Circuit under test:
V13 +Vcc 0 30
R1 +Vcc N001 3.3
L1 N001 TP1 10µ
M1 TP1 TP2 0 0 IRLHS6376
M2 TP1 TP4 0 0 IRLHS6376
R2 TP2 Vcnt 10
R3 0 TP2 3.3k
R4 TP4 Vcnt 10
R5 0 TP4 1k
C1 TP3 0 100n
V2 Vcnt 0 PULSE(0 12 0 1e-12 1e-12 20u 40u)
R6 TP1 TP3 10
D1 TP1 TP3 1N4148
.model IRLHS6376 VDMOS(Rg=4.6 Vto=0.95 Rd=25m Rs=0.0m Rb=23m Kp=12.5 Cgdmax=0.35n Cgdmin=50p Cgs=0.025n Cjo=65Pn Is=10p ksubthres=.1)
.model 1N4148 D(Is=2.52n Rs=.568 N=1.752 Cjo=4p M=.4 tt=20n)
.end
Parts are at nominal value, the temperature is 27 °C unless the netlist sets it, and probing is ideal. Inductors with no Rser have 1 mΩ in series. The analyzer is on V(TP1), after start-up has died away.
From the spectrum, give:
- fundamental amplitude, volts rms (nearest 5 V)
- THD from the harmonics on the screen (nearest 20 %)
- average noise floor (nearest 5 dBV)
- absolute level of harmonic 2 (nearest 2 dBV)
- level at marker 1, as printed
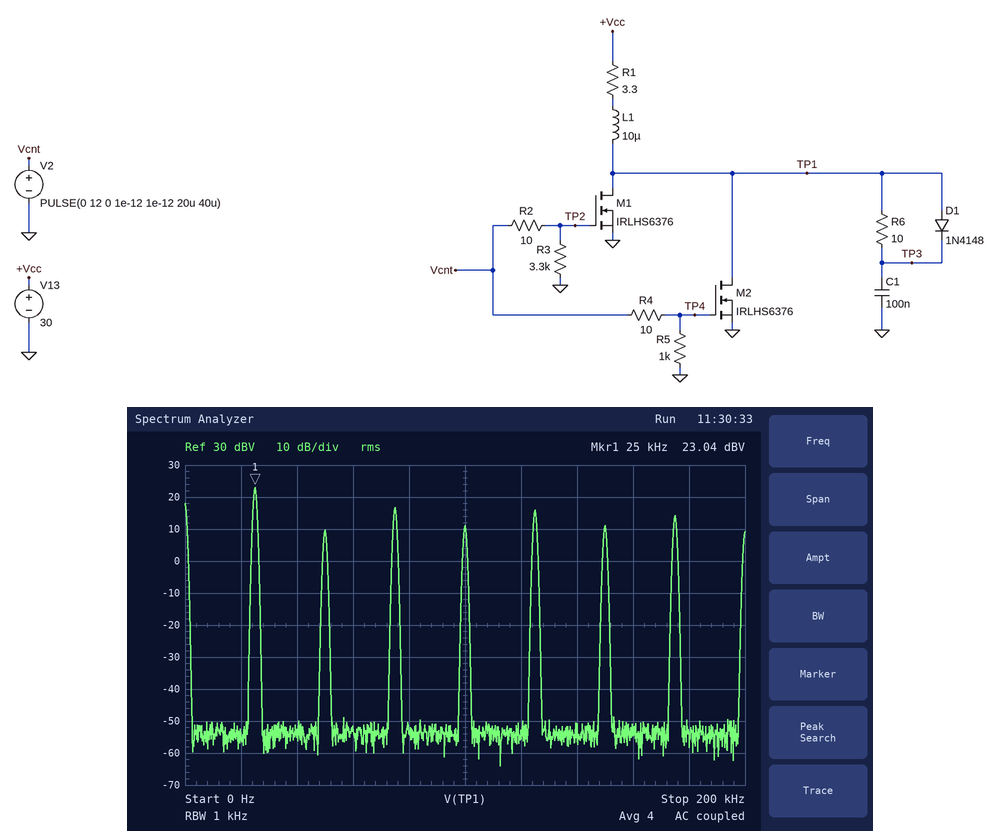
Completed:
15 V
80 %
-55 dBV
10 dBV
23.04 dBV
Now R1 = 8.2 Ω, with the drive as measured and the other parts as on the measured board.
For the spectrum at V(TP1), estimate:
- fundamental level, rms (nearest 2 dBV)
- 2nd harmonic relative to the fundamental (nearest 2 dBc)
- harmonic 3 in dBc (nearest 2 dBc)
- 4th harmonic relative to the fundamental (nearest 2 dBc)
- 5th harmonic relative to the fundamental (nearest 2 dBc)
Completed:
22 dBV
-28 dBc
-8 dBc
-26 dBc
-12 dBc
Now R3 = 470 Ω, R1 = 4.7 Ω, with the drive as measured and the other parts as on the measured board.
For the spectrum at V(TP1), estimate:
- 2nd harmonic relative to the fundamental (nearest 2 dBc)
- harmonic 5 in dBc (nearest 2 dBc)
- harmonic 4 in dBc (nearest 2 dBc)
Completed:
-18 dBc
-10 dBc
-16 dBc
